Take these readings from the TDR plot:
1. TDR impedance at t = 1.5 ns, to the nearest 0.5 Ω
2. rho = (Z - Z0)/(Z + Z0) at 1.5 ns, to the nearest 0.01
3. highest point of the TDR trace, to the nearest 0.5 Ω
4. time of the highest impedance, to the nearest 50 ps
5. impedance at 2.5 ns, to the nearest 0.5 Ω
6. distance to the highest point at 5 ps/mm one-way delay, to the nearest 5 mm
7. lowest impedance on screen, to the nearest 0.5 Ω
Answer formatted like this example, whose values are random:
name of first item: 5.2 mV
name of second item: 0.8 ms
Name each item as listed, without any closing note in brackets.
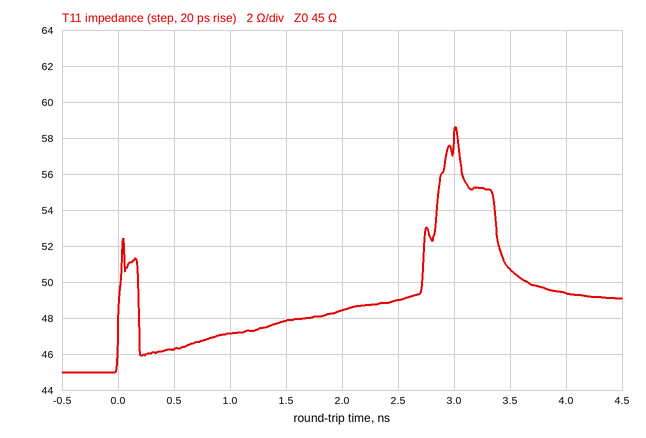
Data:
TDR impedance at t = 1.5 ns, to the nearest 0.5 Ω: 48.0 Ω
rho = (Z - Z0)/(Z + Z0) at 1.5 ns, to the nearest 0.01: +0.03
highest point of the TDR trace, to the nearest 0.5 Ω: 58.5 Ω
time of the highest impedance, to the nearest 50 ps: 3.00 ns
impedance at 2.5 ns, to the nearest 0.5 Ω: 49.0 Ω
distance to the highest point at 5 ps/mm one-way delay, to the nearest 5 mm: 300 mm
lowest impedance on screen, to the nearest 0.5 Ω: 45.0 Ω
